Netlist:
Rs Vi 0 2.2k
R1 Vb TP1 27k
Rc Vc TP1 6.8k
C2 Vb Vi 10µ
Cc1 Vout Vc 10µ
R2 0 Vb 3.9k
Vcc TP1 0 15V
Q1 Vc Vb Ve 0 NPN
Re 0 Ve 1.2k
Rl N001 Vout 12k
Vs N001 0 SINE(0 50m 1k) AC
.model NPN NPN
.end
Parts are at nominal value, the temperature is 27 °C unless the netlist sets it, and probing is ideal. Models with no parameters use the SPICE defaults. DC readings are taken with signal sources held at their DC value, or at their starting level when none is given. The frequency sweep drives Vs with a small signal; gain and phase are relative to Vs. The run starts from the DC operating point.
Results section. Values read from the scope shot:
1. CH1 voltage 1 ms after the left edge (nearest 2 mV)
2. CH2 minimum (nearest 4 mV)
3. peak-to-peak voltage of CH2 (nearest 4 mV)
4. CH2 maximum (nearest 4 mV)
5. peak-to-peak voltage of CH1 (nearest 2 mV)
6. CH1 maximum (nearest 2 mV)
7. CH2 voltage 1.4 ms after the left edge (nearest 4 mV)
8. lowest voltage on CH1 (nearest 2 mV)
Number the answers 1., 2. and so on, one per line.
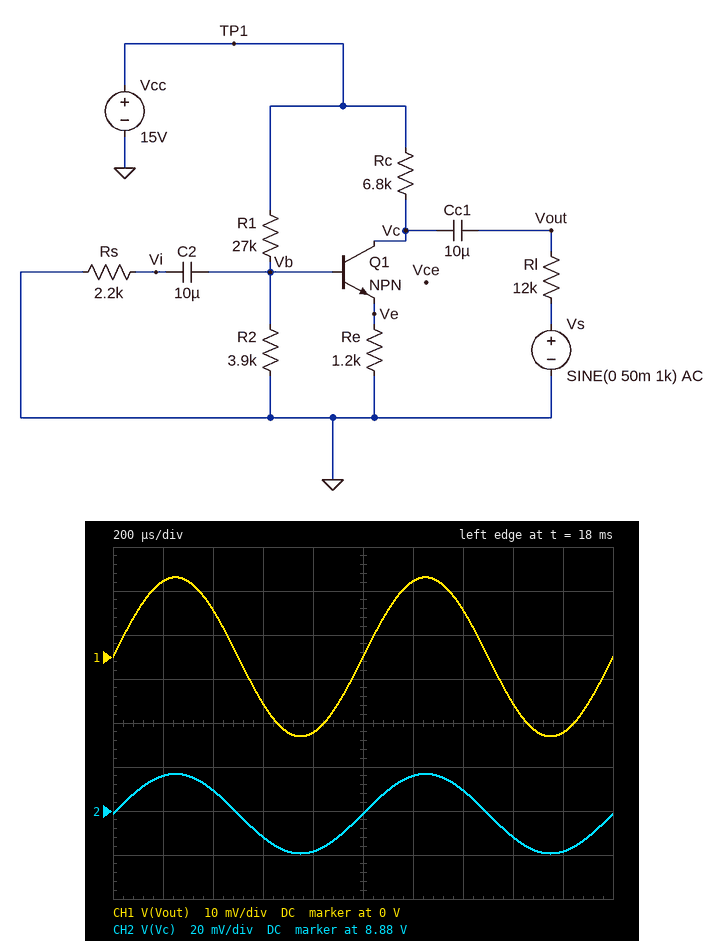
1. 0 V
2. 8.860 V
3. 36 mV
4. 8.896 V
5. 36 mV
6. 18 mV
7. 8.888 V
8. -18 mV
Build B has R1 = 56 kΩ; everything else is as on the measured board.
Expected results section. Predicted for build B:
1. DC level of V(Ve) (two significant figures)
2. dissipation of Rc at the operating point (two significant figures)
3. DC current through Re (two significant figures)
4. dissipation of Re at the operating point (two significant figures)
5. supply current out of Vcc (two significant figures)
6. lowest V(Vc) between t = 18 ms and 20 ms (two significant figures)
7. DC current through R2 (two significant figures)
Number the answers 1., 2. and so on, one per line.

1. 240 mV
2. 260 µW
3. 200 µA
4. 47 µW
5. 450 µA
6. 14 V
7. 250 µA
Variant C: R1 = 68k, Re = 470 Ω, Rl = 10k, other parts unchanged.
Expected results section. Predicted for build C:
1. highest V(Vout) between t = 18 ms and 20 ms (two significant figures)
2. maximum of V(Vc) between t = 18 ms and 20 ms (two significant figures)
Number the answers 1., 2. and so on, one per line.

1. 20 mV
2. 14 V
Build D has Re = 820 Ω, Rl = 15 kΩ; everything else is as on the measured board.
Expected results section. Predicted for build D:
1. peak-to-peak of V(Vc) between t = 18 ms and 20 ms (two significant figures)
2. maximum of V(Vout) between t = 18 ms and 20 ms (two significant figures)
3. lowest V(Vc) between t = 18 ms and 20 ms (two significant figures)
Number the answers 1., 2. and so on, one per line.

1. 31 mV
2. 16 mV
3. 6.2 V
